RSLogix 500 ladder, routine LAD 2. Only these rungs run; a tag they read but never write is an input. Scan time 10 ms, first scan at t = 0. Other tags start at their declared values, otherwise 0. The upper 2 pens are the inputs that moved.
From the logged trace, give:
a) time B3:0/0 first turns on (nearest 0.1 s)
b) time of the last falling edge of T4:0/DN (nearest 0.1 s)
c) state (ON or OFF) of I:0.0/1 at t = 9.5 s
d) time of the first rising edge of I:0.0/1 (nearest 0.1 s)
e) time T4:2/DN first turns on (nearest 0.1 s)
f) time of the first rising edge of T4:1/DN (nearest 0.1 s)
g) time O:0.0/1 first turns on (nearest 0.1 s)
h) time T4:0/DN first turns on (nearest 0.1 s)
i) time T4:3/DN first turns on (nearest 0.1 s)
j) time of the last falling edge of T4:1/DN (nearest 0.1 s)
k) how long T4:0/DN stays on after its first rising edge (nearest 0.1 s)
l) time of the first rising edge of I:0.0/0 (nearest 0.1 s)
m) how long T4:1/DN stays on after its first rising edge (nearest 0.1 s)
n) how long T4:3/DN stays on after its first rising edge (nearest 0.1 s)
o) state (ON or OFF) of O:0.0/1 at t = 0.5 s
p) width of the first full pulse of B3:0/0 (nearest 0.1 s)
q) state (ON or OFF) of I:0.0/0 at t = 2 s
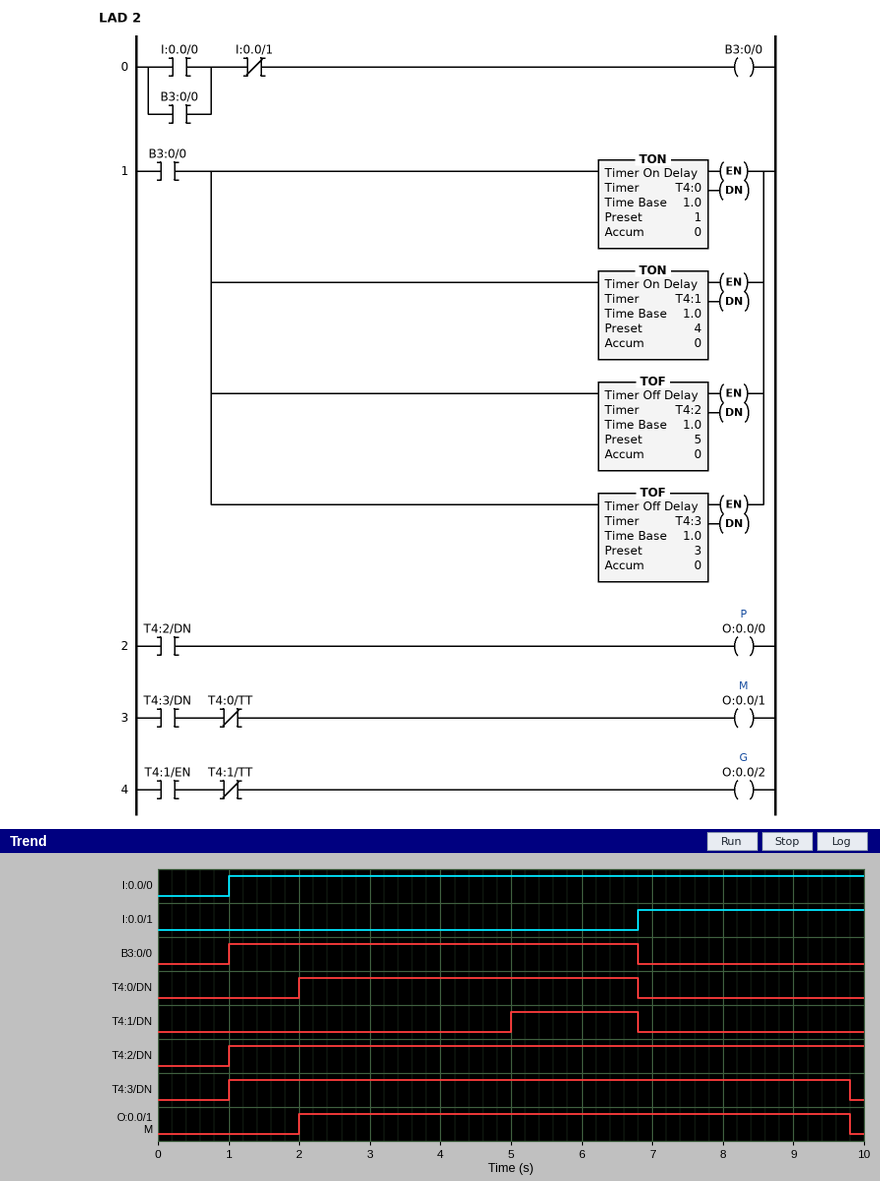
1.0 s
6.8 s
ON
6.8 s
1.0 s
5.0 s
2.0 s
2.0 s
1.0 s
6.8 s
4.8 s
1.0 s
1.8 s
8.8 s
OFF
5.8 s
ON
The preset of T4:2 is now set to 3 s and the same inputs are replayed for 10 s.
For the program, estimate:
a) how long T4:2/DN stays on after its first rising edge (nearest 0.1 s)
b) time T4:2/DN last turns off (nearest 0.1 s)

8.8 s
9.8 s
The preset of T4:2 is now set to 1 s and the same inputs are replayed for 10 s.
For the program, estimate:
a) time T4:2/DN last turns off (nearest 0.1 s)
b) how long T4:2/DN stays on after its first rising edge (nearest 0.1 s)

7.8 s
6.8 s
